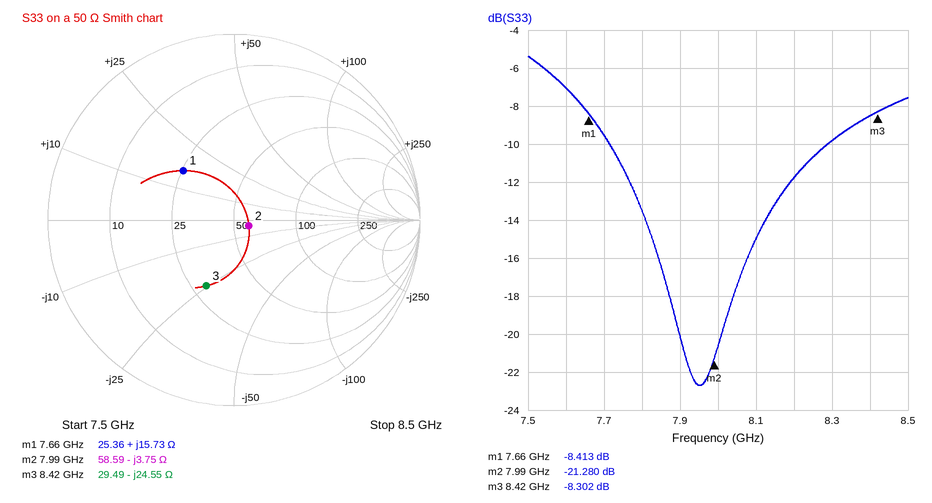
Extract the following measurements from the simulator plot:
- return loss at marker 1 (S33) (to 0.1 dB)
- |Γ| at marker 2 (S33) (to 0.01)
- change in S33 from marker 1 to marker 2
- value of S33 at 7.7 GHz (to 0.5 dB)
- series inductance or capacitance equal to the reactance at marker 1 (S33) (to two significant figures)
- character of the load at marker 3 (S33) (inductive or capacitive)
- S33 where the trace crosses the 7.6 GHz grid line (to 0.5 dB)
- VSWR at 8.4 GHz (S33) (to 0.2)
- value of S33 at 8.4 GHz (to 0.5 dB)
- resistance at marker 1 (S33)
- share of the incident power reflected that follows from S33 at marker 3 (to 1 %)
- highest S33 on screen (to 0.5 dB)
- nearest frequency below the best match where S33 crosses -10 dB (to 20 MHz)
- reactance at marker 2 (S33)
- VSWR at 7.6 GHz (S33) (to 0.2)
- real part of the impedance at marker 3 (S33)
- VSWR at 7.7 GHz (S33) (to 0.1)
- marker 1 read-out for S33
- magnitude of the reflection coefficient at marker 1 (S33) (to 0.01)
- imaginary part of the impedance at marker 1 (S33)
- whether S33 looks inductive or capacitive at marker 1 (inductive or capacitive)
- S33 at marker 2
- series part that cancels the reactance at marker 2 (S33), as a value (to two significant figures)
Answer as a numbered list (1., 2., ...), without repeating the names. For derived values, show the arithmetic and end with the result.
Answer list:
1. 8.4 dB
2. 0.09
3. -21.28 − (-8.413) = -12.867 dB
4. -9.5 dB
5. L = 15.73 Ω/(2π × 7.66 GHz) ≈ 327 pH, so 330 pH to two significant figures
6. capacitive
7. -7.0 dB
8. |Γ| = 10^(-8.5/20) = 0.3758; VSWR = (1 + 0.3758)/(1 − 0.3758) ≈ 2.2
9. -8.5 dB
10. 25.36 Ω
11. 10^(-8.302/10) ≈ 15 %
12. -5.5 dB
13. 7.72 GHz
14. -3.75 Ω
15. |Γ| = 10^(-7/20) = 0.4467; VSWR = (1 + 0.4467)/(1 − 0.4467) ≈ 2.6
16. 29.49 Ω
17. |Γ| = 10^(-9.5/20) = 0.3350; VSWR = (1 + 0.3350)/(1 − 0.3350) ≈ 2.0
18. -8.413 dB
19. 10^(-8.413/20) ≈ 0.38
20. +15.73 Ω
21. inductive
22. -21.280 dB
23. L = 3.75 Ω/(2π × 7.99 GHz) ≈ 75 pH
